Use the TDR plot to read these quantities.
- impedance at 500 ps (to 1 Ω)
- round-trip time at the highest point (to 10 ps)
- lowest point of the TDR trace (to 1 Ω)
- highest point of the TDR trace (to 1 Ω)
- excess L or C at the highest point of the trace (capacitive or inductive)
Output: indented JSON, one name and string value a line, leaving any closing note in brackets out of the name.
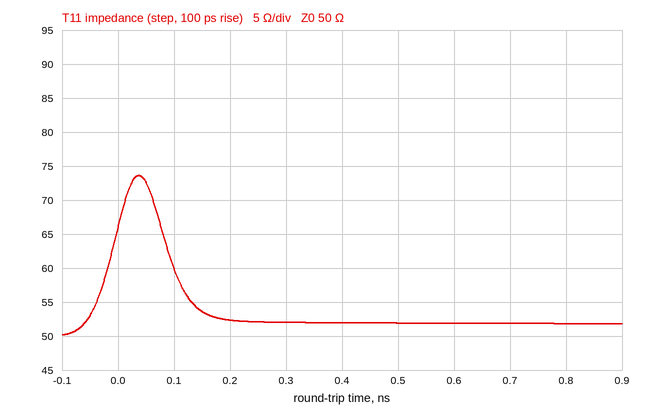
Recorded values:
{
  "impedance at 500 ps": "52 Ω",
  "round-trip time at the highest point": "40 ps",
  "lowest point of the TDR trace": "50 Ω",
  "highest point of the TDR trace": "74 Ω",
  "excess L or C at the highest point of the trace": "inductive"
}
